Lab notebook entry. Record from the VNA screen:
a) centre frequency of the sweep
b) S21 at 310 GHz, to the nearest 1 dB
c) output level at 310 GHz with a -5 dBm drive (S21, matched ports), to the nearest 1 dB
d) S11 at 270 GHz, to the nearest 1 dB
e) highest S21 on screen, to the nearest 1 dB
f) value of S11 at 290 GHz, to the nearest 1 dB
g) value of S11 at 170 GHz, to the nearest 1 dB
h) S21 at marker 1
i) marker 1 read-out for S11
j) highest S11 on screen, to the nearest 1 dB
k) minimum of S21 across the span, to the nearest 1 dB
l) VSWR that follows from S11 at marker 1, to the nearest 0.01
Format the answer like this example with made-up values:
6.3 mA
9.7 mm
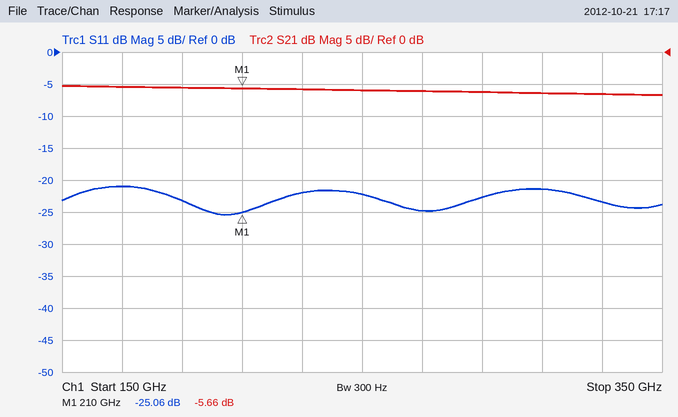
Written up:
250 GHz
-6 dB
-11 dBm
-25 dB
-5 dB
-23 dB
-21 dB
-5.66 dB
-25.06 dB
-21 dB
-7 dB
1.12
